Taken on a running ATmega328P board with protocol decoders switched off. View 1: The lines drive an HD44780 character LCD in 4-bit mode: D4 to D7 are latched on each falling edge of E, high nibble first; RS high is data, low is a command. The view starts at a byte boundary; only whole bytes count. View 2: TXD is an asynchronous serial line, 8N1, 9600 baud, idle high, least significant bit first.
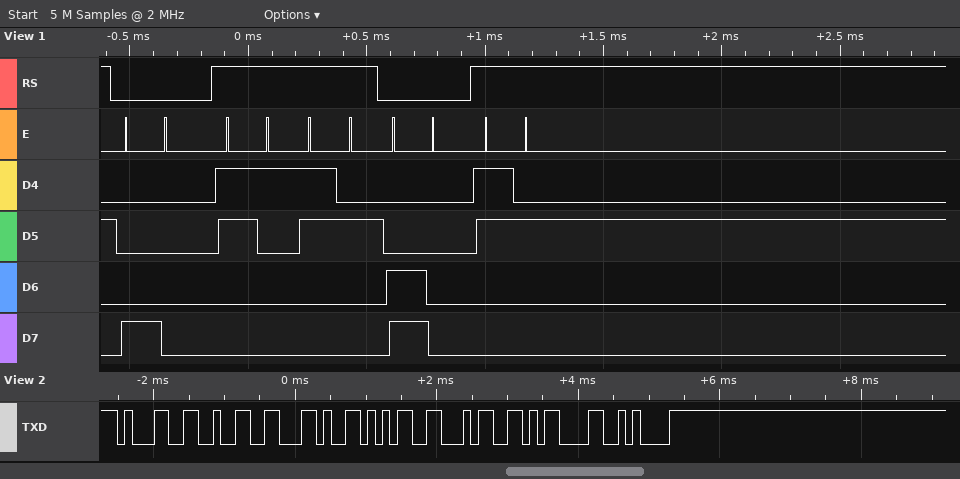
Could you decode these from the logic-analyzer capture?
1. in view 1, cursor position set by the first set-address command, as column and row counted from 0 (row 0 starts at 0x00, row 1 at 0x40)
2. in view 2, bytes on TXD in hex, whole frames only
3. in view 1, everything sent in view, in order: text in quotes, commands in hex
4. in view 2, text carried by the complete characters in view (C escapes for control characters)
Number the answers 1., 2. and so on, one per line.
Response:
1. column 0, row 0
2. 31 32 2C 35 34 0D 0A
3. 0x80 "12" 0xC0 "2"
4. "12,54\r\n"
